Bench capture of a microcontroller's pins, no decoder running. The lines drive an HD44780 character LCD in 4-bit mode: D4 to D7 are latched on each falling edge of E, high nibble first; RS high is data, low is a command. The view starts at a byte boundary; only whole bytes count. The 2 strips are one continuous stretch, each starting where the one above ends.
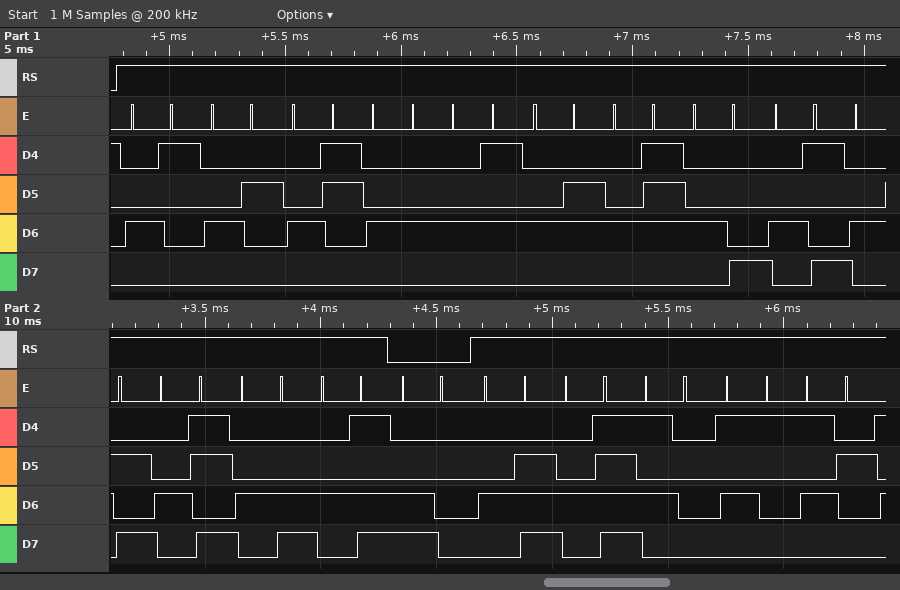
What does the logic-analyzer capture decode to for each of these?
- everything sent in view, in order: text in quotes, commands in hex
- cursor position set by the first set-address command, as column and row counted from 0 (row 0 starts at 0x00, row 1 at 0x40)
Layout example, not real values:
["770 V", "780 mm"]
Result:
["\"ABCDEFGHIJKLM\" 0xC0 \"NOPQR\"", "column 0, row 1"]
